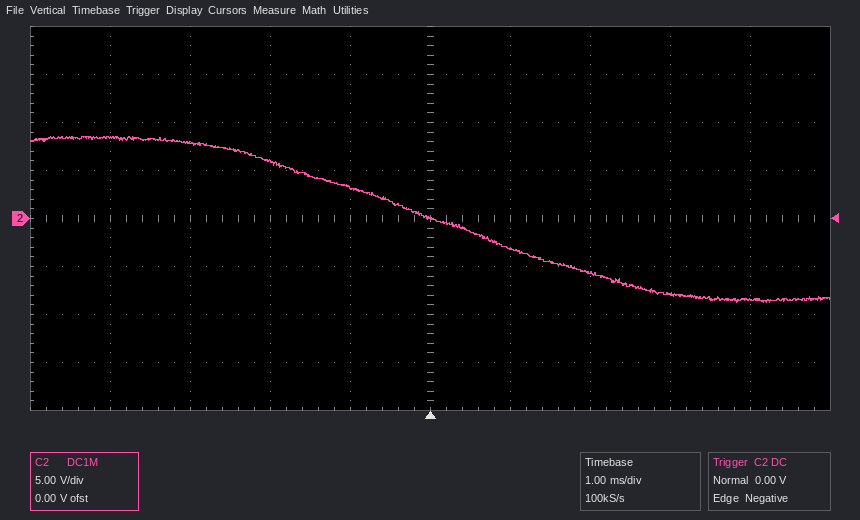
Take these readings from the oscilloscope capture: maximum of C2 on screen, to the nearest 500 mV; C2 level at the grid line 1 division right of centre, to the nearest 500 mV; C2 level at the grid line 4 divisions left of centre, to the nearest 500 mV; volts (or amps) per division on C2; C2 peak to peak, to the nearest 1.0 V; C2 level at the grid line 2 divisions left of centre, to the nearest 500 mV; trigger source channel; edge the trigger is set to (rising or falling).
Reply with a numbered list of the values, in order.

1. 8.5 V
2. -3.0 V
3. 8.5 V
4. 5 V
5. 17.0 V
6. 6.0 V
7. C2
8. falling
